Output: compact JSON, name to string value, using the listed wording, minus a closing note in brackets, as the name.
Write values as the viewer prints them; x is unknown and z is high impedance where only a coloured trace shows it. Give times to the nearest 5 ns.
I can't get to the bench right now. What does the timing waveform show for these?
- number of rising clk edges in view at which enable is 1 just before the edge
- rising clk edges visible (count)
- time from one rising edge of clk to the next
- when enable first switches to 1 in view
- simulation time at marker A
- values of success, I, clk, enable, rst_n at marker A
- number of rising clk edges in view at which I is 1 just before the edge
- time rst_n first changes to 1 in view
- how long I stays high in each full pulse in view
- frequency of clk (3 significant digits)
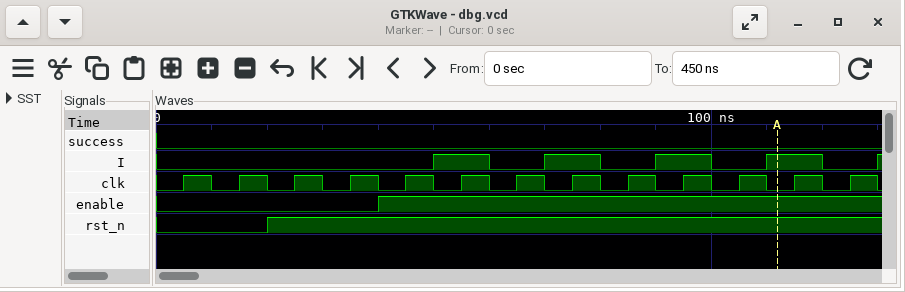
{"number of rising clk edges in view at which enable is 1 just before the edge": "9", "rising clk edges visible": "13", "time from one rising edge of clk to the next": "10 ns", "when enable first switches to 1 in view": "40 ns", "simulation time at marker A": "110 ns", "values of success, I, clk, enable, rst_n at marker A": "success=0, I=1, clk=0, enable=1, rst_n=1", "number of rising clk edges in view at which I is 1 just before the edge": "4", "time rst_n first changes to 1 in view": "20 ns", "how long I stays high in each full pulse in view": "10 ns, 10 ns, 10 ns, 10 ns", "frequency of clk": "100 MHz"}
